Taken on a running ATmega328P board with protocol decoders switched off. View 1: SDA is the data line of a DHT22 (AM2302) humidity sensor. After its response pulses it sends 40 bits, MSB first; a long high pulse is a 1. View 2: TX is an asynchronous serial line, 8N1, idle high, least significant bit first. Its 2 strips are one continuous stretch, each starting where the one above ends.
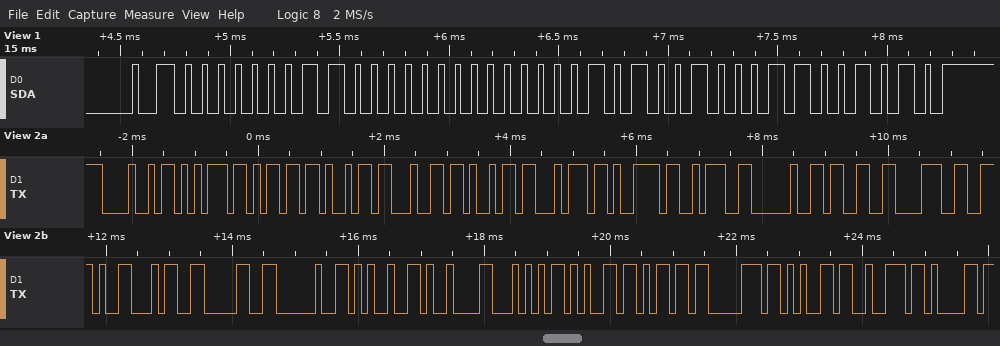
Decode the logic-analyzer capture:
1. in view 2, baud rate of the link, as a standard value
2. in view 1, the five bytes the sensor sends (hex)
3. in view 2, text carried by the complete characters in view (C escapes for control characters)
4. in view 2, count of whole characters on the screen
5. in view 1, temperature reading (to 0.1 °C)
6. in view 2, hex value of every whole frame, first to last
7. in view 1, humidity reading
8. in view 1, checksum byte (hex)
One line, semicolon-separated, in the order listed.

9600 baud; 01 80 01 48 CA; "Humidity: 38.40 %\tTempera"; 25; 32.8 °C; 0x48 0x75 0x6D 0x69 0x64 0x69 0x74 0x79 0x3A 0x20 0x33 0x38 0x2E 0x34 0x30 0x20 0x25 0x09 0x54 0x65 0x6D 0x70 0x65 0x72 0x61; 38.4 %; 0xCA
